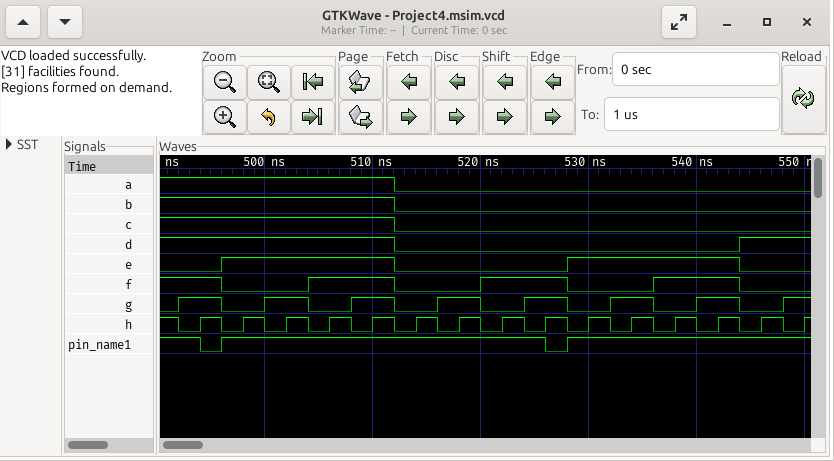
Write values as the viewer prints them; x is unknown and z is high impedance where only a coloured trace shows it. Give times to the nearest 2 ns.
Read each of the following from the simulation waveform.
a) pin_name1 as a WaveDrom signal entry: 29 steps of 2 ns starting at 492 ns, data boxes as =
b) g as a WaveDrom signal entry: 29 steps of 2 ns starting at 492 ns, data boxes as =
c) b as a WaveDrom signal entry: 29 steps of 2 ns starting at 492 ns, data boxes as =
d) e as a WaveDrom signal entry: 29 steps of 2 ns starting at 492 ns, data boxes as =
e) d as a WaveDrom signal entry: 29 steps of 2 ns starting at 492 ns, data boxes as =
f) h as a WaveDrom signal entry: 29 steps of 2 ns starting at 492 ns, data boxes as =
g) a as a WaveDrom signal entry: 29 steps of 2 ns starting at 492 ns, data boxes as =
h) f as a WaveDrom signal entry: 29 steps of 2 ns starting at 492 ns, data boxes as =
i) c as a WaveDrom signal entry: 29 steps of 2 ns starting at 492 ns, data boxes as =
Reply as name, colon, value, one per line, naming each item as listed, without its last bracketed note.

pin_name1 as a WaveDrom signal entry: 29 steps of 2 ns starting at 492 ns, data boxes as =: {name: 'pin_name1', wave: '101..............01..........'}
g as a WaveDrom signal entry: 29 steps of 2 ns starting at 492 ns, data boxes as =: {name: 'g', wave: '1.0.1.0.1.0.1.0.1.0.1.0.1.0.1'}
b as a WaveDrom signal entry: 29 steps of 2 ns starting at 492 ns, data boxes as =: {name: 'b', wave: '1.........0..................'}
e as a WaveDrom signal entry: 29 steps of 2 ns starting at 492 ns, data boxes as =: {name: 'e', wave: '0.1.......0.......1.......0..'}
d as a WaveDrom signal entry: 29 steps of 2 ns starting at 492 ns, data boxes as =: {name: 'd', wave: '1.........0...............1..'}
h as a WaveDrom signal entry: 29 steps of 2 ns starting at 492 ns, data boxes as =: {name: 'h', wave: '01010101010101010101010101010'}
a as a WaveDrom signal entry: 29 steps of 2 ns starting at 492 ns, data boxes as =: {name: 'a', wave: '1.........0..................'}
f as a WaveDrom signal entry: 29 steps of 2 ns starting at 492 ns, data boxes as =: {name: 'f', wave: '1.0...1...0...1...0...1...0..'}
c as a WaveDrom signal entry: 29 steps of 2 ns starting at 492 ns, data boxes as =: {name: 'c', wave: '1.........0..................'}
